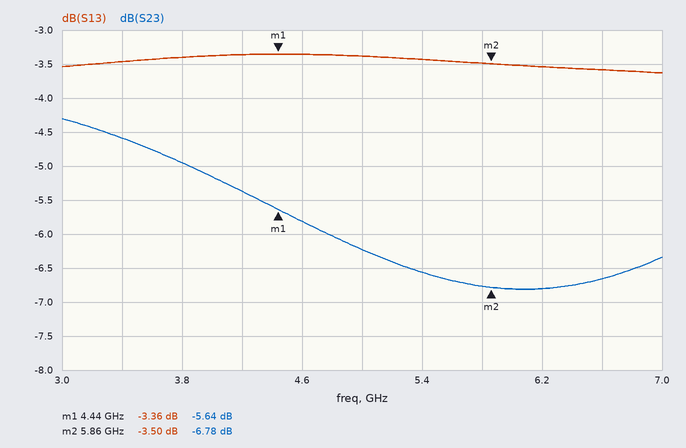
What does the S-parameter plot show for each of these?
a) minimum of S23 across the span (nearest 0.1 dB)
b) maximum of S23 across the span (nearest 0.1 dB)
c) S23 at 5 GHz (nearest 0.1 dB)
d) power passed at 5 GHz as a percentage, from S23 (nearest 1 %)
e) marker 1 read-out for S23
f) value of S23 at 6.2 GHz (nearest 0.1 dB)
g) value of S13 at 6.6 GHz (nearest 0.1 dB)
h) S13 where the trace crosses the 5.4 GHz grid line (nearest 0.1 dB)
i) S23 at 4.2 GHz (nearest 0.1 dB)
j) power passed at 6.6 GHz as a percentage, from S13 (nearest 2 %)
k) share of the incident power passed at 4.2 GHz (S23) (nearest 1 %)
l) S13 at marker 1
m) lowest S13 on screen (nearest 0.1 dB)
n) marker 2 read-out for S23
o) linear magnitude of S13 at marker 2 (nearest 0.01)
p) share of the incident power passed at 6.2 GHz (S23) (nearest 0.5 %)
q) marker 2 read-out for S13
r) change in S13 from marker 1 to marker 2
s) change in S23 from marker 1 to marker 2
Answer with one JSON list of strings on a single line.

["-6.8 dB", "-4.3 dB", "-6.2 dB", "24 %", "-5.64 dB", "-6.8 dB", "-3.6 dB", "-3.4 dB", "-5.4 dB", "44 %", "29 %", "-3.36 dB", "-3.6 dB", "-6.78 dB", "0.67", "21.0 %", "-3.50 dB", "-0.14 dB", "-1.14 dB"]
